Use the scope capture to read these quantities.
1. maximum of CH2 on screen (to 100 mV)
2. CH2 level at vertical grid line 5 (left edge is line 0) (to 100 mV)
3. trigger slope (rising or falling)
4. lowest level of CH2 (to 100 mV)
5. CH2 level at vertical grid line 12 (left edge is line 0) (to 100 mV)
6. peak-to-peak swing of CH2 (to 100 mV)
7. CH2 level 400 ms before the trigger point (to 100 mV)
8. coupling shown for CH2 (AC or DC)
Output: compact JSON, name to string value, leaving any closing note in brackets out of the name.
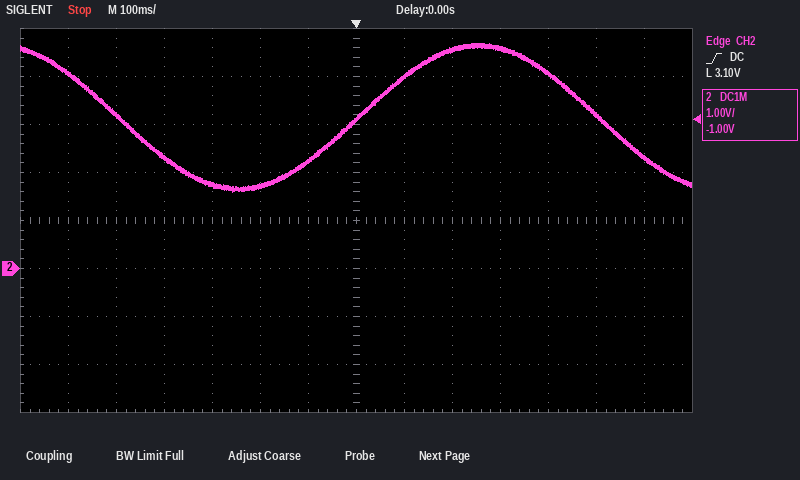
{"maximum of CH2 on screen": "4.7 V", "CH2 level at vertical grid line 5 (left edge is line 0)": "1.7 V", "trigger slope": "rising", "lowest level of CH2": "1.6 V", "CH2 level at vertical grid line 12 (left edge is line 0)": "3.2 V", "peak-to-peak swing of CH2": "3.1 V", "CH2 level 400 ms before the trigger point": "2.3 V", "coupling shown for CH2": "DC"}
